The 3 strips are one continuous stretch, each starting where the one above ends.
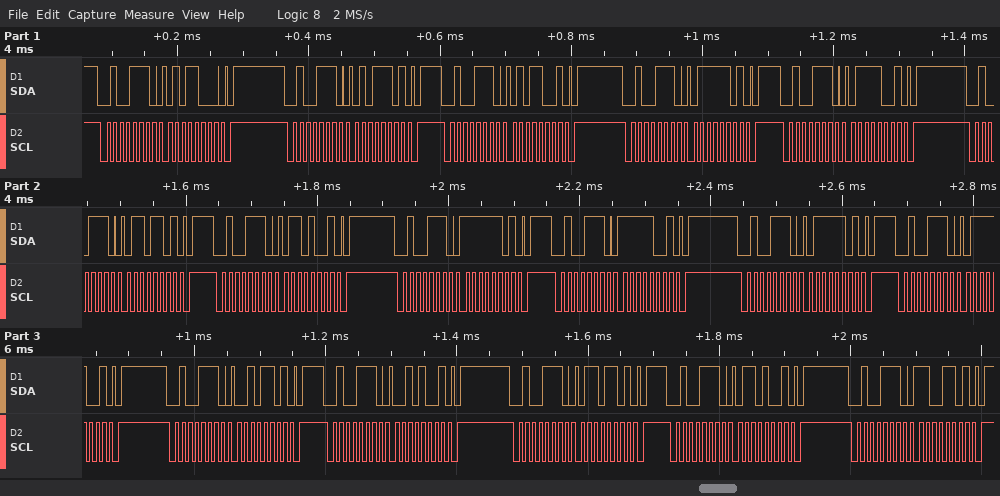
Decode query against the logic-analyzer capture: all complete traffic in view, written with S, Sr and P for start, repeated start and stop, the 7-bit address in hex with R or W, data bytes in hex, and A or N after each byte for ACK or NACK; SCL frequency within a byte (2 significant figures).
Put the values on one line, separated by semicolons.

S 27W A 58 A P S 27W A 5D A P S 27W A 59 A P S 27W A 7D A P S 27W A 79 A P S 27W A 6D A P S 27W A 69 A P S 27W A FD A P S 27W A F9 A P S 27W A 7D A P S 27W A 79 A P S 27W A 2D A P S 27W A 29 A P S 27W A 6D A P S 27W A 69 A P S 27W A CD A P; 100 kHz
